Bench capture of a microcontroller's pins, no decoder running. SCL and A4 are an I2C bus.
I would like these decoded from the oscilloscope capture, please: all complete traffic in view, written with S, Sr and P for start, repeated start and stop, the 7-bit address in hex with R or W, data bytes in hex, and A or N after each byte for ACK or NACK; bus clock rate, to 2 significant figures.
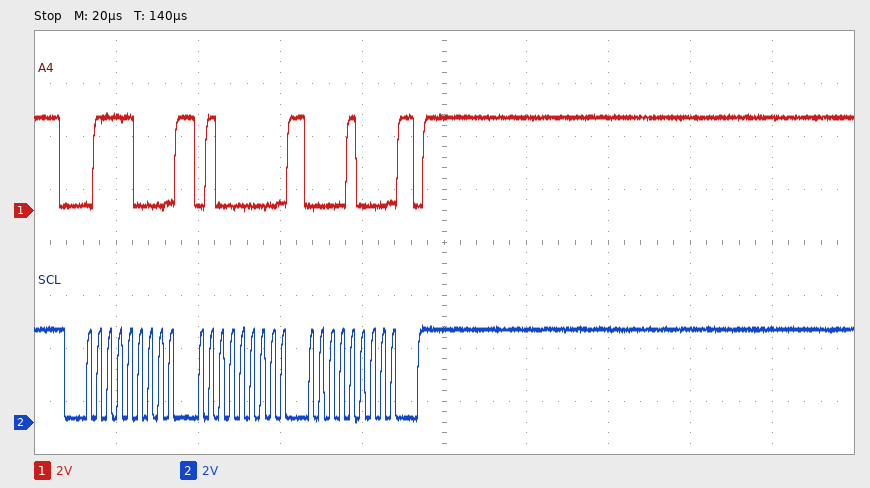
S 3CW A 40 A 08 A P
400 kHz
